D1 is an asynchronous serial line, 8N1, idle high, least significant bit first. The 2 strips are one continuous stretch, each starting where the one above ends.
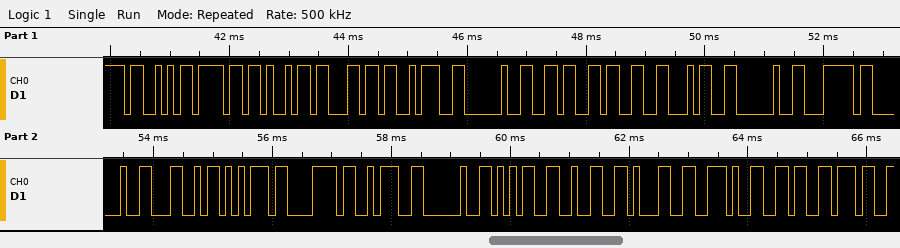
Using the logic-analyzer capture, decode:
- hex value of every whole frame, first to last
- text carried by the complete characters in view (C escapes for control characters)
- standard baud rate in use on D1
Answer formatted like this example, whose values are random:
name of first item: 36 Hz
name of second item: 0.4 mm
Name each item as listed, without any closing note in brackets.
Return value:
hex value of every whole frame, first to last: 53 6F 69 6C 3A 20 36 33 34 20 7C 20 4C 75 78 3A 20 35 32 31 2E 36 37
text carried by the complete characters in view: "Soil: 634 | Lux: 521.67"
standard baud rate in use on D1: 9600 baud
